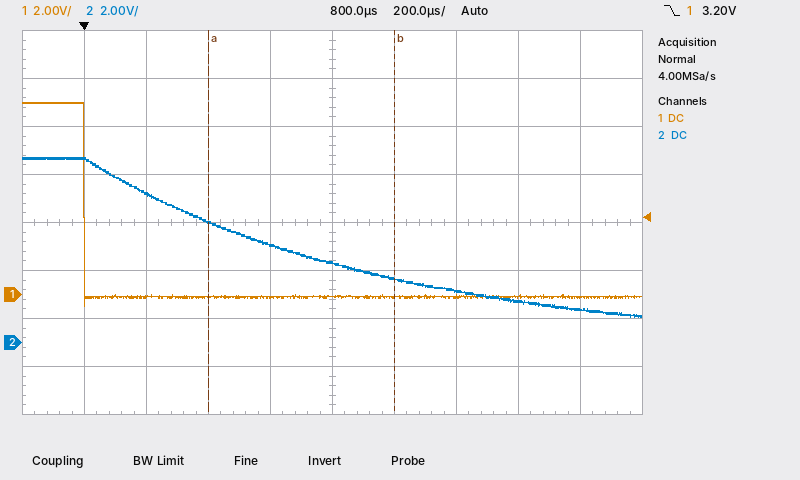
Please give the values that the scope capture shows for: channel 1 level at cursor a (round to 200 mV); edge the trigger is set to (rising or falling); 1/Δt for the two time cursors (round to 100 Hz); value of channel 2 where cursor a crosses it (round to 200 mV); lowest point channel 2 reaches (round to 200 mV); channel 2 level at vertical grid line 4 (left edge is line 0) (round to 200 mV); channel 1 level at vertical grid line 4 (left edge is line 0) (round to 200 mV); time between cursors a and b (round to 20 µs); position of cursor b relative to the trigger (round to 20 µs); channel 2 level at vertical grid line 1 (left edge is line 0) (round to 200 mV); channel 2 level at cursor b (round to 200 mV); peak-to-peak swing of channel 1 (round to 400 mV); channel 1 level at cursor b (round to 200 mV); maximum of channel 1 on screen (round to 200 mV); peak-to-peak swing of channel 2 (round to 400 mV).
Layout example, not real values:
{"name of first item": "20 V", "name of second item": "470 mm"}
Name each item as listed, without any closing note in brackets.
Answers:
{"channel 1 level at cursor a": "-200 mV", "edge the trigger is set to": "falling", "1/Δt for the two time cursors": "1.7 kHz", "value of channel 2 where cursor a crosses it": "5.0 V", "lowest point channel 2 reaches": "1.0 V", "channel 2 level at vertical grid line 4 (left edge is line 0)": "4.0 V", "channel 1 level at vertical grid line 4 (left edge is line 0)": "-200 mV", "time between cursors a and b": "600 µs", "position of cursor b relative to the trigger": "+1.00 ms", "channel 2 level at vertical grid line 1 (left edge is line 0)": "7.6 V", "channel 2 level at cursor b": "2.6 V", "peak-to-peak swing of channel 1": "8.4 V", "channel 1 level at cursor b": "-200 mV", "maximum of channel 1 on screen": "8.0 V", "peak-to-peak swing of channel 2": "6.8 V"}
